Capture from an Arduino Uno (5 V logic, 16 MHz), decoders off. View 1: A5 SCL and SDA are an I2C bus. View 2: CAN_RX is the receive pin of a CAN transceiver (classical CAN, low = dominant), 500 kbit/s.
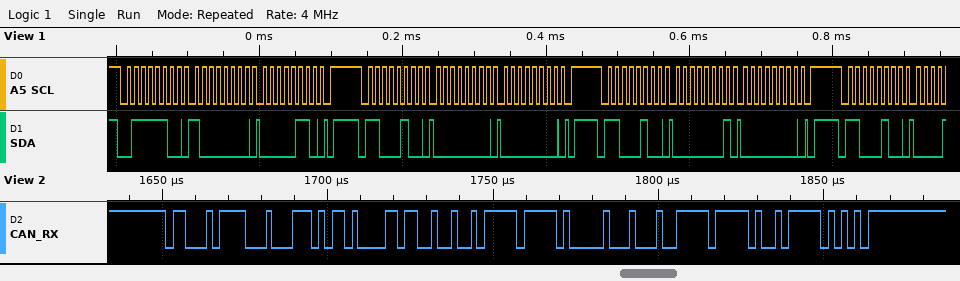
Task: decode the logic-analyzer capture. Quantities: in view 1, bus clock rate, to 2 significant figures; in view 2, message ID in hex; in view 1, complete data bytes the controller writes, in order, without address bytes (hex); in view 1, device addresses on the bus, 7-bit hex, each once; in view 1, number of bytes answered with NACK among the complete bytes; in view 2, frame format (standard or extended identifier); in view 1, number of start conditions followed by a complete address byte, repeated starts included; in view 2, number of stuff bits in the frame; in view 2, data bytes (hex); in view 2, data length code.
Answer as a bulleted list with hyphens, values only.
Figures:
- 100 kHz
- 0x62F
- 80 06 00 00 01 00
- 0x3E 0x62
- 0
- standard
- 4
- 6
- EB 43 64 97 FF 00 89 FF
- 8
